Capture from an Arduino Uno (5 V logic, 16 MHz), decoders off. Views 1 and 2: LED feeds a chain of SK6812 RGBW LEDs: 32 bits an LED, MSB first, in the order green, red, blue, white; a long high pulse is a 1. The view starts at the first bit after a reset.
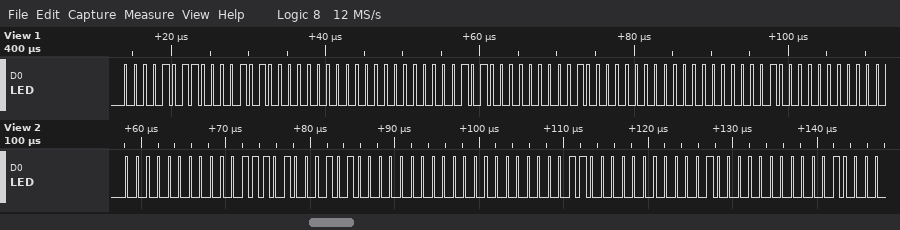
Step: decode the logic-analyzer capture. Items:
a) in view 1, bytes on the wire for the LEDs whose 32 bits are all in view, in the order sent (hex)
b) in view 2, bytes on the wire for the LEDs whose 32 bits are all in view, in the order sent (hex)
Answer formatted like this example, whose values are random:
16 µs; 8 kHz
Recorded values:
0B 0A 00 00 14 01 00 00; 00 1D 14 00 00 30 01 00
